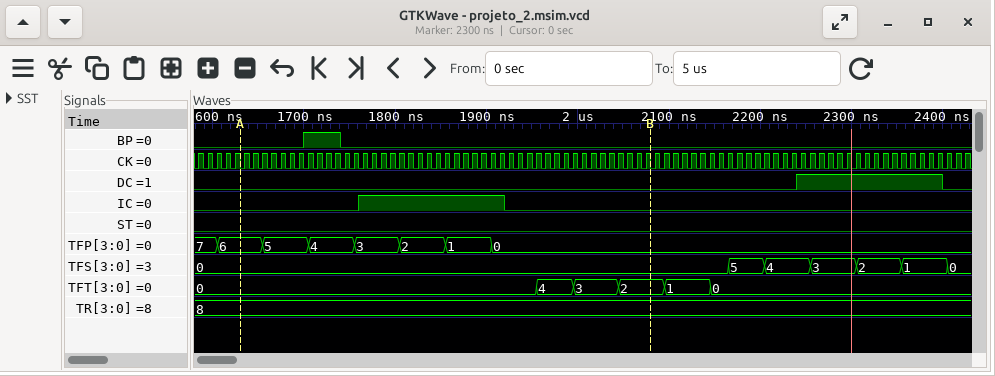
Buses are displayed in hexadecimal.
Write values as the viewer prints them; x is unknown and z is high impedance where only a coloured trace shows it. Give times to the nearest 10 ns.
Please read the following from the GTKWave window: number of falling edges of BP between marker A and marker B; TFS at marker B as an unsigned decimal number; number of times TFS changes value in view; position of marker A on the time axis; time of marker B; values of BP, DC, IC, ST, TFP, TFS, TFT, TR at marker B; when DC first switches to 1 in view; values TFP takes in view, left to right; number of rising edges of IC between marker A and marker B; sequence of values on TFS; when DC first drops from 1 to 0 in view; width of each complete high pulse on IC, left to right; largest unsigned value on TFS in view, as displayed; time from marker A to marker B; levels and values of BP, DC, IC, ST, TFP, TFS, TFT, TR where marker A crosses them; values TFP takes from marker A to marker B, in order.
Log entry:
1
0
6
1630 ns
2080 ns
BP=0, DC=0, IC=0, ST=0, TFP=0, TFS=0, TFT=2, TR=8
2240 ns
7, 6, 5, 4, 3, 2, 1, 0
1
0, 5, 4, 3, 2, 1, 0
2400 ns
160 ns
5
450 ns
BP=0, DC=0, IC=0, ST=0, TFP=6, TFS=0, TFT=0, TR=8
6, 5, 4, 3, 2, 1, 0
